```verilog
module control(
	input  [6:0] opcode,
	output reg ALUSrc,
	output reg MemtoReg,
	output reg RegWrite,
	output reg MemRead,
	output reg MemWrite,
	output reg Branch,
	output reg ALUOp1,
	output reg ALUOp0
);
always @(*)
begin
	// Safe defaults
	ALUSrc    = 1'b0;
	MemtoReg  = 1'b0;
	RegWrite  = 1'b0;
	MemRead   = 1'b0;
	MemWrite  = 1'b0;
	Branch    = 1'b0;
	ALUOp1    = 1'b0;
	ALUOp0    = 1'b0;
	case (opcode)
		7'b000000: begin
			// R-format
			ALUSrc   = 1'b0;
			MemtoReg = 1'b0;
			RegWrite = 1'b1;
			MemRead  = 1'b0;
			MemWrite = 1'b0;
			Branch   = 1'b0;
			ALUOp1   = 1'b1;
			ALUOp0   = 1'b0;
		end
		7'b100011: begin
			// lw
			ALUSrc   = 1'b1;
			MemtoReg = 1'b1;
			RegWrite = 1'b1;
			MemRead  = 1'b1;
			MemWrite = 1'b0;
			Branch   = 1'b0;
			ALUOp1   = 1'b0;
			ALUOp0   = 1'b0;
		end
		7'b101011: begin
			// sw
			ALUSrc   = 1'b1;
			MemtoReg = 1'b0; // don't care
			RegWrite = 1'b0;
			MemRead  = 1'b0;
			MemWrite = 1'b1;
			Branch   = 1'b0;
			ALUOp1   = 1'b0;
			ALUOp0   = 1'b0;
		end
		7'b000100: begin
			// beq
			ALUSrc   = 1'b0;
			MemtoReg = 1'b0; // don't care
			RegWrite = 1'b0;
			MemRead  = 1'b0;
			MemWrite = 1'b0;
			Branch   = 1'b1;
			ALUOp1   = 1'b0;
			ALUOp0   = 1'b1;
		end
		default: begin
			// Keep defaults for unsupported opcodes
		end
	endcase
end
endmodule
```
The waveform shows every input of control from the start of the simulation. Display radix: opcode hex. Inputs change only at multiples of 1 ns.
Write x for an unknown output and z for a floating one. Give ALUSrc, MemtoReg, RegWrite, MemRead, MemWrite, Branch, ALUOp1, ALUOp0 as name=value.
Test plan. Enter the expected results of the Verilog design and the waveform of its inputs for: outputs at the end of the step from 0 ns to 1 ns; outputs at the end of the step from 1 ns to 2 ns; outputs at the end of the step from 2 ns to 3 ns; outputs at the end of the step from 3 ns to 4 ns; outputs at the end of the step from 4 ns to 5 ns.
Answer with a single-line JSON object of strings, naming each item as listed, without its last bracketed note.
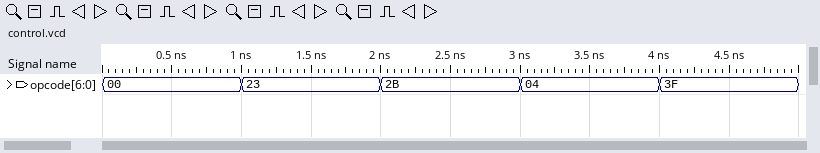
{"outputs at the end of the step from 0 ns to 1 ns": "ALUSrc=0, MemtoReg=0, RegWrite=1, MemRead=0, MemWrite=0, Branch=0, ALUOp1=1, ALUOp0=0", "outputs at the end of the step from 1 ns to 2 ns": "ALUSrc=1, MemtoReg=1, RegWrite=1, MemRead=1, MemWrite=0, Branch=0, ALUOp1=0, ALUOp0=0", "outputs at the end of the step from 2 ns to 3 ns": "ALUSrc=1, MemtoReg=0, RegWrite=0, MemRead=0, MemWrite=1, Branch=0, ALUOp1=0, ALUOp0=0", "outputs at the end of the step from 3 ns to 4 ns": "ALUSrc=0, MemtoReg=0, RegWrite=0, MemRead=0, MemWrite=0, Branch=1, ALUOp1=0, ALUOp0=1", "outputs at the end of the step from 4 ns to 5 ns": "ALUSrc=0, MemtoReg=0, RegWrite=0, MemRead=0, MemWrite=0, Branch=0, ALUOp1=0, ALUOp0=0"}
